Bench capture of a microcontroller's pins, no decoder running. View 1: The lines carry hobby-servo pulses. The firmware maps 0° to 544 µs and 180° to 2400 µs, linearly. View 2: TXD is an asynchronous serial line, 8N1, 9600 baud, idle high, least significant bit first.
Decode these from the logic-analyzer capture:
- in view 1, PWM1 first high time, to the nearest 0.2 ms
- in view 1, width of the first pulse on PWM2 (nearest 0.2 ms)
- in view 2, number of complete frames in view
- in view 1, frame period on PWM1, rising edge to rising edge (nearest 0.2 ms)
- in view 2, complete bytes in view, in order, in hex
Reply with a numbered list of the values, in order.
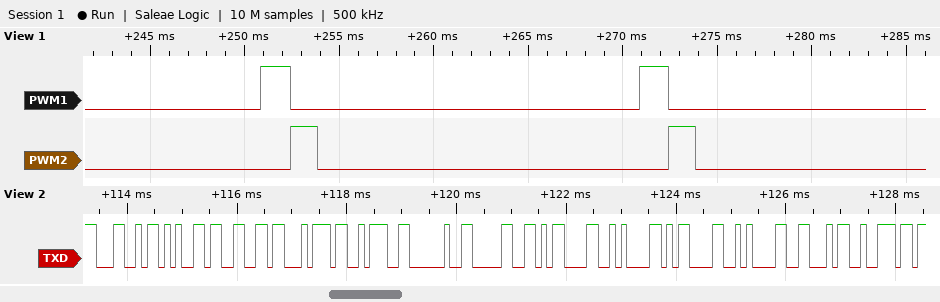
1. 1.6 ms
2. 1.4 ms
3. 13
4. 20.0 ms
5. 4C 65 66 74 3A 20 30 0D 0A 0D 0A 46 72
